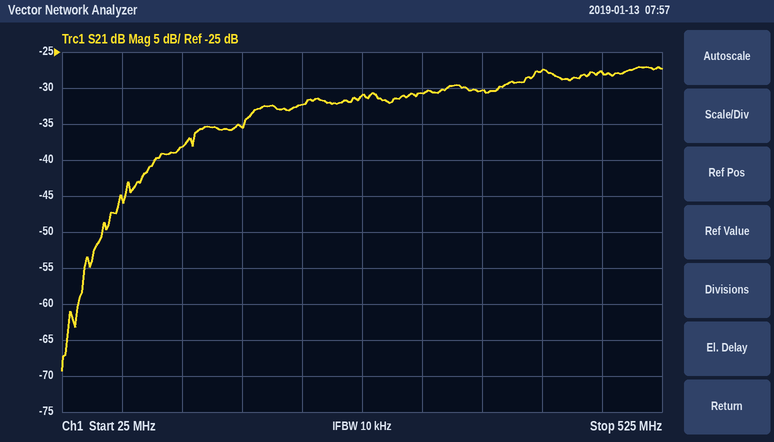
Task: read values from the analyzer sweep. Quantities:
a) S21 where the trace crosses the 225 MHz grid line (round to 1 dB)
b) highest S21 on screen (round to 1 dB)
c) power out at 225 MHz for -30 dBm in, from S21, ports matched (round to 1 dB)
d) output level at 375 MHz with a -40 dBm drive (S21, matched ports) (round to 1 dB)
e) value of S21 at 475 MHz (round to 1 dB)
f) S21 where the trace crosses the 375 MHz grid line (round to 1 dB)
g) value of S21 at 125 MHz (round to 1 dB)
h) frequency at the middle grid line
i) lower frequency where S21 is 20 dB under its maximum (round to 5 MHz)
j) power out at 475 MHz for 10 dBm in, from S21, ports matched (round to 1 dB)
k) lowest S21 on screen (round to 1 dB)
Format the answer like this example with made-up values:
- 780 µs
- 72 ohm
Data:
- -32 dB
- -27 dB
- -62 dBm
- -70 dBm
- -28 dB
- -30 dB
- -38 dB
- 275 MHz
- 70 MHz
- -18 dBm
- -69 dB
